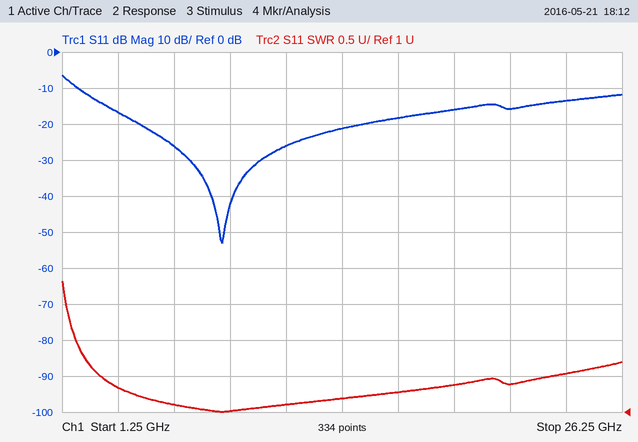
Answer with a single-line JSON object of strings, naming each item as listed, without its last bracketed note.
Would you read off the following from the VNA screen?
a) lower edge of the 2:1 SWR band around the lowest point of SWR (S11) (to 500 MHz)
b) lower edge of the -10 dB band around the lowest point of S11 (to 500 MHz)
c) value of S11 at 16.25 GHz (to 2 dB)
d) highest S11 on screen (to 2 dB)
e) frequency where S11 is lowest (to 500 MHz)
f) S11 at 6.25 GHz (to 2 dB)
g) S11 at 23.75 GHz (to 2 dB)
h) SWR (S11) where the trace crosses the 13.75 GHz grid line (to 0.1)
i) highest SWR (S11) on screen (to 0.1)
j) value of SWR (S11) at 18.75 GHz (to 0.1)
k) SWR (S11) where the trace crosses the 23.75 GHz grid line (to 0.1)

{"lower edge of the 2:1 SWR band around the lowest point of SWR (S11)": "2.0 GHz", "lower edge of the -10 dB band around the lowest point of S11": "2.0 GHz", "value of S11 at 16.25 GHz": "-18 dB", "highest S11 on screen": "-6 dB", "frequency where S11 is lowest": "8.5 GHz", "S11 at 6.25 GHz": "-26 dB", "S11 at 23.75 GHz": "-14 dB", "SWR (S11) where the trace crosses the 13.75 GHz grid line": "1.2", "highest SWR (S11) on screen": "2.8", "value of SWR (S11) at 18.75 GHz": "1.4", "SWR (S11) where the trace crosses the 23.75 GHz grid line": "1.5"}
